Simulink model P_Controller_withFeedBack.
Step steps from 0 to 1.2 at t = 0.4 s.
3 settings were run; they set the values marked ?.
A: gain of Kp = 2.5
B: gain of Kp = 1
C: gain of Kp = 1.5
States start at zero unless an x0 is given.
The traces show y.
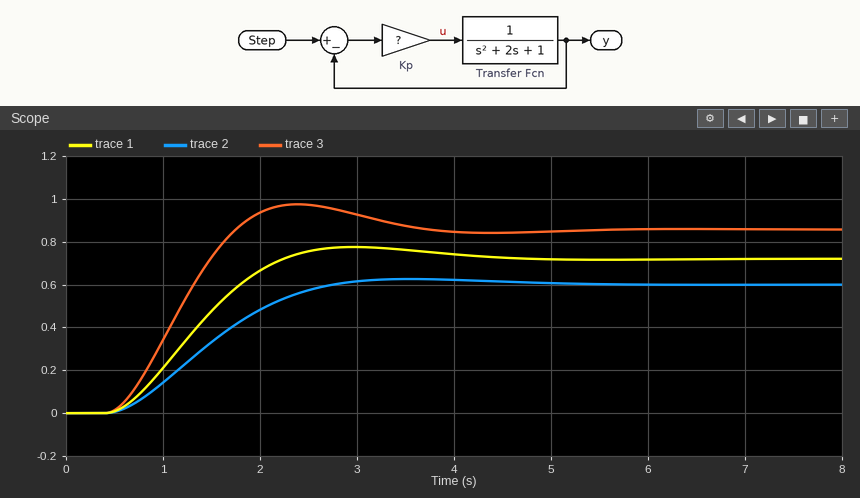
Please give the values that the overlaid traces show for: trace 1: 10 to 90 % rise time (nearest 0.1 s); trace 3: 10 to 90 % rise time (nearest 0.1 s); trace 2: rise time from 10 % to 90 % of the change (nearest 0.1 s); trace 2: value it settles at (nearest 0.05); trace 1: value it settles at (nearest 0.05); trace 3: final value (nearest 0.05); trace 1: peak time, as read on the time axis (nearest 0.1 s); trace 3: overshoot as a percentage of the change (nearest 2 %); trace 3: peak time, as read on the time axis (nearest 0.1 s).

1.2 s
0.9 s
1.5 s
0.60
0.70
0.85
3.0 s
14 %
2.4 s
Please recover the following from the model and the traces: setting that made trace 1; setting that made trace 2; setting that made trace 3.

C
B
A
